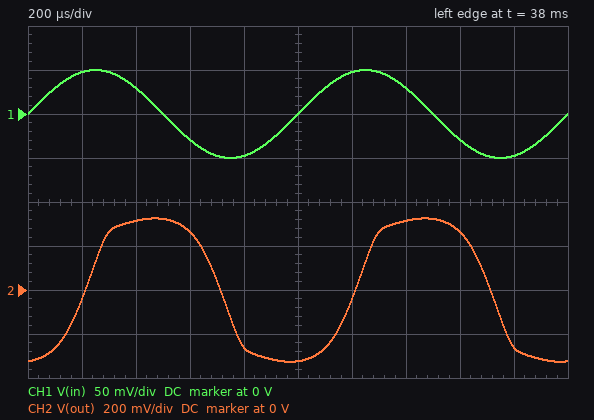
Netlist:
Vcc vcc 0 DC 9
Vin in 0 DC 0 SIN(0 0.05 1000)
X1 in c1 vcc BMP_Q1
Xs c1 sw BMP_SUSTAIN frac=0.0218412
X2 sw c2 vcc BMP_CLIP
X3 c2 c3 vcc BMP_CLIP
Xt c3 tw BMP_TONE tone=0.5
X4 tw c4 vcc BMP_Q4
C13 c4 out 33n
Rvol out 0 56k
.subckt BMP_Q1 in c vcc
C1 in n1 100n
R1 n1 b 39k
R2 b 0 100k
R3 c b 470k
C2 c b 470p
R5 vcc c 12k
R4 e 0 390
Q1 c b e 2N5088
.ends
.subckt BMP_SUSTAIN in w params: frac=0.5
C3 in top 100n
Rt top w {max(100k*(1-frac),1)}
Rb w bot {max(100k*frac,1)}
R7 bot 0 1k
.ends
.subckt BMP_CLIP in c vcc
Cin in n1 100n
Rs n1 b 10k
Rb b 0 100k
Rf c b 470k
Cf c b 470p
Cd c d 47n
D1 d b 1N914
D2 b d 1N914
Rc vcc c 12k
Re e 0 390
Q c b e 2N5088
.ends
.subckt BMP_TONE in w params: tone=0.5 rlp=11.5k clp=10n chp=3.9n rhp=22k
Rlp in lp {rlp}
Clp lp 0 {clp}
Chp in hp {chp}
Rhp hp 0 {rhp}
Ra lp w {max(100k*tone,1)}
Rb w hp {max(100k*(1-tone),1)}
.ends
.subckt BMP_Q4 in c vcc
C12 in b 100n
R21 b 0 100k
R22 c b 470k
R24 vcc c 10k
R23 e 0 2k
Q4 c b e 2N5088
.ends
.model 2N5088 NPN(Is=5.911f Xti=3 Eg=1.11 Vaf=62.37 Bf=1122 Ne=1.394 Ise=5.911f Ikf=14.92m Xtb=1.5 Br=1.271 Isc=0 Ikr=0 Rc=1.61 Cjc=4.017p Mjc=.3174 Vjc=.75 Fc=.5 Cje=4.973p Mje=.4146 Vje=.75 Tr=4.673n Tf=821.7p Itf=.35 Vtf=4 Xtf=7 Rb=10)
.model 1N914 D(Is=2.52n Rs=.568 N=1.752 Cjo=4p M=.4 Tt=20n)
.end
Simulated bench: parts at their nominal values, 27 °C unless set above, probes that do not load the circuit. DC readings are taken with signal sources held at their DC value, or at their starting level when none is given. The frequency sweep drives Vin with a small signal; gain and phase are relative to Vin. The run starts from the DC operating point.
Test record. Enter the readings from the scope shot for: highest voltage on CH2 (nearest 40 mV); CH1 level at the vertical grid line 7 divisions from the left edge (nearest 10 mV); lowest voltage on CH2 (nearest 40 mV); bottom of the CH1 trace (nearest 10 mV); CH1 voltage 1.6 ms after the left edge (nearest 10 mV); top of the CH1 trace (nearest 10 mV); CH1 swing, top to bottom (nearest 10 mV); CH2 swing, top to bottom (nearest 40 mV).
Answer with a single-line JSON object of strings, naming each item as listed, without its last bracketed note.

{"highest voltage on CH2": "320 mV", "CH1 level at the vertical grid line 7 divisions from the left edge": "30 mV", "lowest voltage on CH2": "-320 mV", "bottom of the CH1 trace": "-50 mV", "CH1 voltage 1.6 ms after the left edge": "-30 mV", "top of the CH1 trace": "50 mV", "CH1 swing, top to bottom": "100 mV", "CH2 swing, top to bottom": "640 mV"}
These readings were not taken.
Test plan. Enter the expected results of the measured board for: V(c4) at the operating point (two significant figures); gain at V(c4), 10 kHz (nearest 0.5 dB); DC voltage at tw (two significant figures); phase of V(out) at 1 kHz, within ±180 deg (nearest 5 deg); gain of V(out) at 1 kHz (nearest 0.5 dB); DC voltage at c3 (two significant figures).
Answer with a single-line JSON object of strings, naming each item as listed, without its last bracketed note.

{"V(c4) at the operating point": "6.5 V", "gain at V(c4), 10 kHz": "-15.5 dB", "DC voltage at tw": "2.5 V", "phase of V(out) at 1 kHz, within ±180 deg": "-90 deg", "gain of V(out) at 1 kHz": "22.5 dB", "DC voltage at c3": "4.6 V"}
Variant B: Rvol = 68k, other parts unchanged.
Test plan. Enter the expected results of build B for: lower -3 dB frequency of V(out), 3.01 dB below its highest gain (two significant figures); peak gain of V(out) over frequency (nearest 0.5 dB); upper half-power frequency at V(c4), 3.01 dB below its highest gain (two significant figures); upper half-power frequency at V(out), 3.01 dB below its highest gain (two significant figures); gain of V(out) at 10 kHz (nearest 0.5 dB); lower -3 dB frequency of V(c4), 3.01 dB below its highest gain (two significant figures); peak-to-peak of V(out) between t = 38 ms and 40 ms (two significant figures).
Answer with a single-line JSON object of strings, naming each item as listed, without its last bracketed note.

{"lower -3 dB frequency of V(out), 3.01 dB below its highest gain": "93 Hz", "peak gain of V(out) over frequency": "29.0 dB", "upper half-power frequency at V(c4), 3.01 dB below its highest gain": "650 Hz", "upper half-power frequency at V(out), 3.01 dB below its highest gain": "680 Hz", "gain of V(out) at 10 kHz": "-15.0 dB", "lower -3 dB frequency of V(c4), 3.01 dB below its highest gain": "71 Hz", "peak-to-peak of V(out) between t = 38 ms and 40 ms": "670 mV"}
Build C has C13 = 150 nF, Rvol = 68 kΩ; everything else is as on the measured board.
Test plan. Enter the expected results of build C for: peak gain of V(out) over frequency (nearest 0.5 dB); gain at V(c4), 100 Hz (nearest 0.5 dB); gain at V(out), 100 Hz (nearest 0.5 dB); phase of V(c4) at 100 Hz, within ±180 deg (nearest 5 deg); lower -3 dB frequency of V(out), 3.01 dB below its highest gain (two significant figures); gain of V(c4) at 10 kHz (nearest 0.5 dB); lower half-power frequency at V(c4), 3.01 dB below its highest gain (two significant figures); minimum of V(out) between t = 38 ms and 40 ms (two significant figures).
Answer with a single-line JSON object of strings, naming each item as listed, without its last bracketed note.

{"peak gain of V(out) over frequency": "29.0 dB", "gain at V(c4), 100 Hz": "28.0 dB", "gain at V(out), 100 Hz": "27.5 dB", "phase of V(c4) at 100 Hz, within ±180 deg": "75 deg", "lower -3 dB frequency of V(out), 3.01 dB below its highest gain": "76 Hz", "gain of V(c4) at 10 kHz": "-15.0 dB", "lower half-power frequency at V(c4), 3.01 dB below its highest gain": "74 Hz", "minimum of V(out) between t = 38 ms and 40 ms": "-340 mV"}
